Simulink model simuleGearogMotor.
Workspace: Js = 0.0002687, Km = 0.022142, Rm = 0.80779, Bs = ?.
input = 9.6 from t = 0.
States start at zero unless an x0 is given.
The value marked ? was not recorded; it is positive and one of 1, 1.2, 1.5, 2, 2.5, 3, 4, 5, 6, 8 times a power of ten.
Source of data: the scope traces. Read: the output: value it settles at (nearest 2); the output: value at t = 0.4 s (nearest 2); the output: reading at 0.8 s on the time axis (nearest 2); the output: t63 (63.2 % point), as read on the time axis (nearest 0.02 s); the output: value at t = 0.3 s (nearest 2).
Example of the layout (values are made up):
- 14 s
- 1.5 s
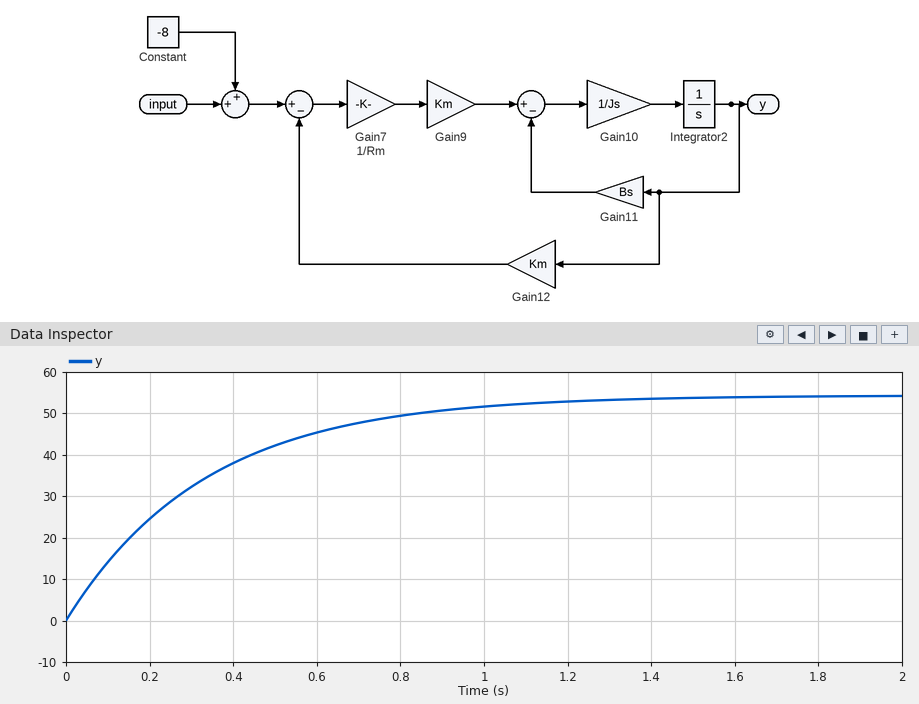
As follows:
- 54
- 38
- 50
- 0.34 s
- 32
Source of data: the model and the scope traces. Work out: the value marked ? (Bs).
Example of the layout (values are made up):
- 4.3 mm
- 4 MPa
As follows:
- 0.0002
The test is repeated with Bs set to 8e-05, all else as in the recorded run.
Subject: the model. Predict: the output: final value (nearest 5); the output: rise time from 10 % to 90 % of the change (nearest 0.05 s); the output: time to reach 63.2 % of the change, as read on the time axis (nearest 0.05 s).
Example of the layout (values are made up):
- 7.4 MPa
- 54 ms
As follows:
- 65
- 0.85 s
- 0.40 s
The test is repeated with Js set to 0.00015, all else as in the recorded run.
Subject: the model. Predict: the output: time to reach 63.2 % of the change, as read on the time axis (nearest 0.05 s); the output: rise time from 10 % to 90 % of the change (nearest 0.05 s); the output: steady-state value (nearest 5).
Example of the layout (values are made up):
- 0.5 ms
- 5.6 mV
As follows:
- 0.20 s
- 0.40 s
- 55
